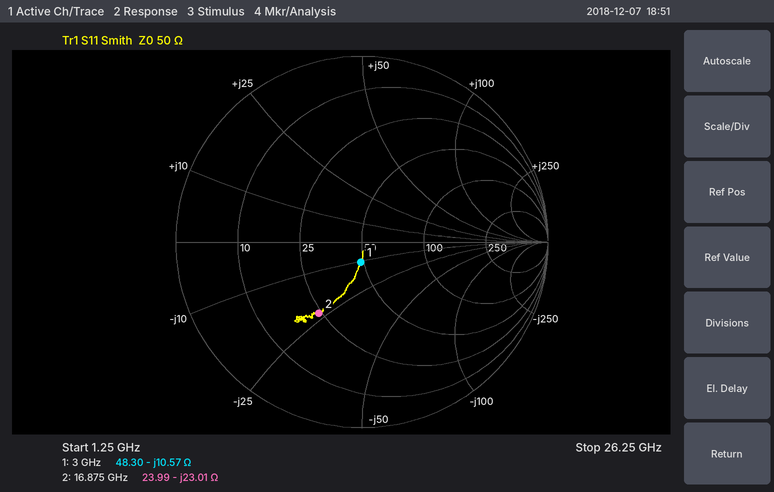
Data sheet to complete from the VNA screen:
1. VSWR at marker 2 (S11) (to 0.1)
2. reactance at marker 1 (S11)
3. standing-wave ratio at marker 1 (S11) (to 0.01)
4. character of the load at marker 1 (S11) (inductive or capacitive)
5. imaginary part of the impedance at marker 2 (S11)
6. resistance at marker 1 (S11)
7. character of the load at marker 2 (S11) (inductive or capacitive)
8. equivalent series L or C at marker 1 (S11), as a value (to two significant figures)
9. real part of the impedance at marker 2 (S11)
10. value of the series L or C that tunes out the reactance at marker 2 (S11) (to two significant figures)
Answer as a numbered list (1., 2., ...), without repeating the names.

1. 2.6
2. -10.57 Ω
3. 1.24
4. capacitive
5. -23.01 Ω
6. 48.30 Ω
7. capacitive
8. 5.0 pF
9. 23.99 Ω
10. 220 pH
